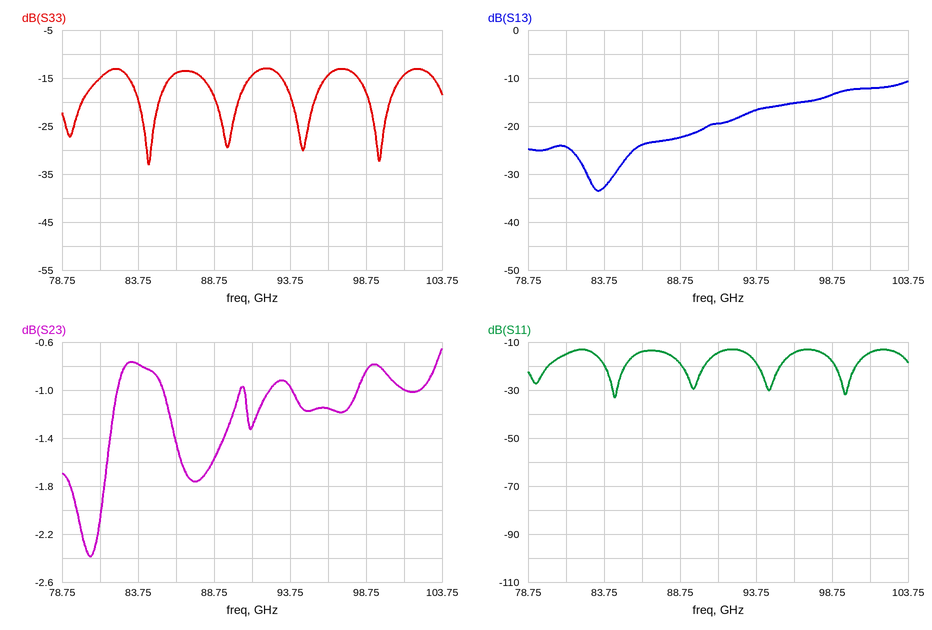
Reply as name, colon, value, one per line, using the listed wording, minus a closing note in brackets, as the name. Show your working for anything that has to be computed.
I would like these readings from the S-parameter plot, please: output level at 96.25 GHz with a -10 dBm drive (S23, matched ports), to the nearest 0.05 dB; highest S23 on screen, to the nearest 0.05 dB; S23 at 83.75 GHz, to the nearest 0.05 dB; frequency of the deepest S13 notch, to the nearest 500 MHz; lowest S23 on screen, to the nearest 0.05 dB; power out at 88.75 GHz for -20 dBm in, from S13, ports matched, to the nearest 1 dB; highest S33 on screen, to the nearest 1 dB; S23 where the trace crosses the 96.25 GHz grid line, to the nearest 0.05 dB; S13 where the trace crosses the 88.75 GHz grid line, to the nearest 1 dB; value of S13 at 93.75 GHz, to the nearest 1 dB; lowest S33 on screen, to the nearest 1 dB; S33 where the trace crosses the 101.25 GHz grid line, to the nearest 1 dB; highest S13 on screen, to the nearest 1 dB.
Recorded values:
output level at 96.25 GHz with a -10 dBm drive (S23, matched ports), to the nearest 0.05 dB: -10 dBm + (-1.15 dB) = -11.15 dBm
highest S23 on screen, to the nearest 0.05 dB: -0.65 dB
S23 at 83.75 GHz, to the nearest 0.05 dB: -0.80 dB
frequency of the deepest S13 notch, to the nearest 500 MHz: 83.5 GHz
lowest S23 on screen, to the nearest 0.05 dB: -2.40 dB
power out at 88.75 GHz for -20 dBm in, from S13, ports matched, to the nearest 1 dB: -20 dBm + (-22 dB) = -42 dBm
highest S33 on screen, to the nearest 1 dB: -13 dB
S23 where the trace crosses the 96.25 GHz grid line, to the nearest 0.05 dB: -1.15 dB
S13 where the trace crosses the 88.75 GHz grid line, to the nearest 1 dB: -22 dB
value of S13 at 93.75 GHz, to the nearest 1 dB: -17 dB
lowest S33 on screen, to the nearest 1 dB: -33 dB
S33 where the trace crosses the 101.25 GHz grid line, to the nearest 1 dB: -14 dB
highest S13 on screen, to the nearest 1 dB: -11 dB
